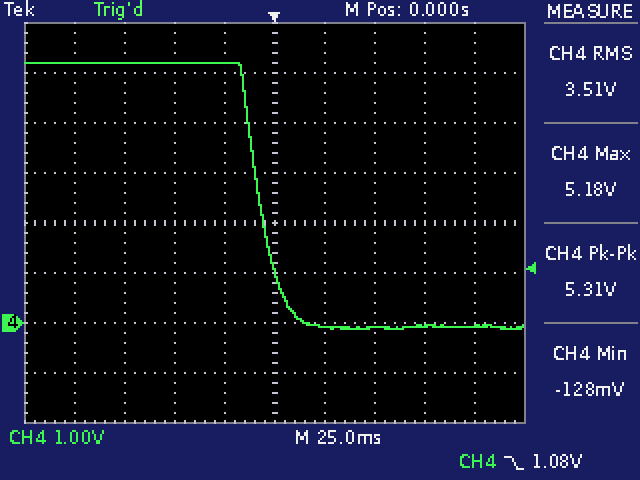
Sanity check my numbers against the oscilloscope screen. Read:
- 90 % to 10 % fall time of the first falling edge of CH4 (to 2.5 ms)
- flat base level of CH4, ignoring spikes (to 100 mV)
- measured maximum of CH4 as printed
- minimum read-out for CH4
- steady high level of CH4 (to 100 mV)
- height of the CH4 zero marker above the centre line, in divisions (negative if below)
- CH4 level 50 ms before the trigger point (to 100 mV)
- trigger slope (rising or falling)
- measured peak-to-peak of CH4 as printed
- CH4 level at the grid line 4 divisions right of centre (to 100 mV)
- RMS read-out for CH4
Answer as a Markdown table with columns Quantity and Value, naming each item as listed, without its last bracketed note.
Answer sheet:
| Quantity | Value |
|---|---|
| 90 % to 10 % fall time of the first falling edge of CH4 | 20.0 ms |
| flat base level of CH4, ignoring spikes | -100 mV |
| measured maximum of CH4 as printed | 5.18 V |
| minimum read-out for CH4 | -128 mV |
| steady high level of CH4 | 5.2 V |
| height of the CH4 zero marker above the centre line, in divisions | -2.0 div |
| CH4 level 50 ms before the trigger point | 5.2 V |
| trigger slope | falling |
| measured peak-to-peak of CH4 as printed | 5.31 V |
| CH4 level at the grid line 4 divisions right of centre | -100 mV |
| RMS read-out for CH4 | 3.51 V |
